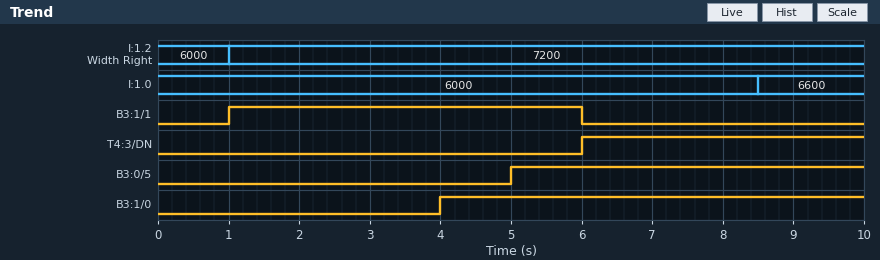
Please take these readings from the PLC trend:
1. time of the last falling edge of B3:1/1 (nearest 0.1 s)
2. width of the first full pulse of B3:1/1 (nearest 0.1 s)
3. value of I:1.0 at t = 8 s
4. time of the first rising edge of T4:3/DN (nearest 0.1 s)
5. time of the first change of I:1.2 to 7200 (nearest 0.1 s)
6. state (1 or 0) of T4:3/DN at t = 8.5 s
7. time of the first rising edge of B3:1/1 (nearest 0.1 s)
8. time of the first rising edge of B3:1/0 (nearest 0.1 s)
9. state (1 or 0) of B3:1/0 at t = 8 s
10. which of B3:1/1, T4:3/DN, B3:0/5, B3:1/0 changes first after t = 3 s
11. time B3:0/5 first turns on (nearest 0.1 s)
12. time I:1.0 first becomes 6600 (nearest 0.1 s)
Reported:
6.0 s
5.0 s
6000
6.0 s
1.0 s
1
1.0 s
4.0 s
1
B3:1/0
5.0 s
8.5 s
